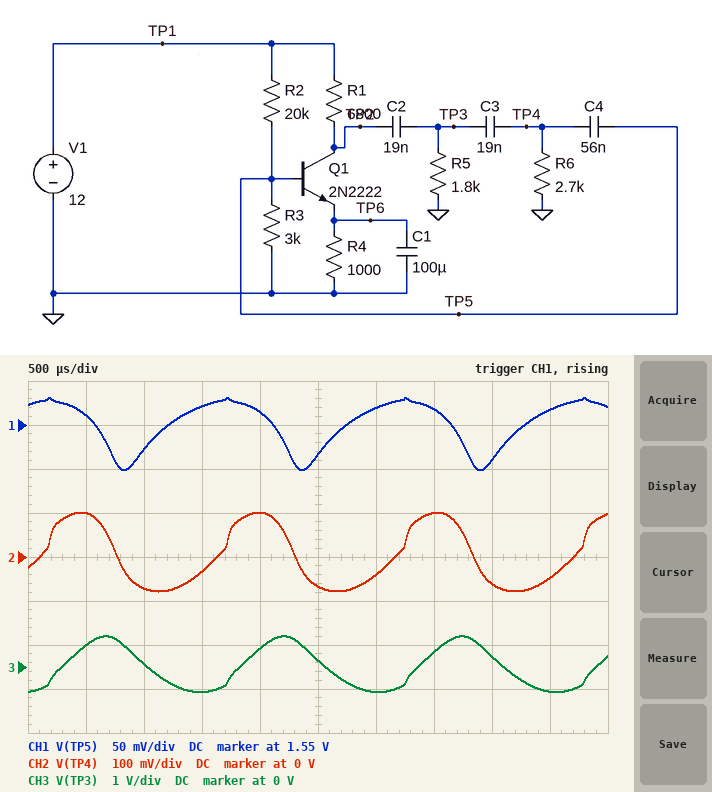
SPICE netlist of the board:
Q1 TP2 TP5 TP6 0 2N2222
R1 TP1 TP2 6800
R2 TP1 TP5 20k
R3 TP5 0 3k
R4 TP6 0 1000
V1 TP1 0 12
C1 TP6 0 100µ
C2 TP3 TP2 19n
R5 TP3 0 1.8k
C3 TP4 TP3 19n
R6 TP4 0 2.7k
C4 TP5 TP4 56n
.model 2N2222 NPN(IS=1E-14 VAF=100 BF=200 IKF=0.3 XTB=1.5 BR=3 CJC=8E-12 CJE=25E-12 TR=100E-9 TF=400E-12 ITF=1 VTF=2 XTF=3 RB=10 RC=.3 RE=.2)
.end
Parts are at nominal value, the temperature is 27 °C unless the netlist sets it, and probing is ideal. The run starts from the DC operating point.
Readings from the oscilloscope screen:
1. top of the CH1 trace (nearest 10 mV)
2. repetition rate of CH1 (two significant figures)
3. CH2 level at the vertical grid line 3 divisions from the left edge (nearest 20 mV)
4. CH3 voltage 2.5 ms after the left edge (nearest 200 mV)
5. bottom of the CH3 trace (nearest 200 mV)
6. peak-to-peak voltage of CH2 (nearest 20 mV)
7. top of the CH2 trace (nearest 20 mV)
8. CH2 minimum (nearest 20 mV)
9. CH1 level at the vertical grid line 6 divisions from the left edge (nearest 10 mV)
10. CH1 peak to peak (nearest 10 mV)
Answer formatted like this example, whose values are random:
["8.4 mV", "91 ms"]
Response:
["1.58 V", "650 Hz", "-40 mV", "200 mV", "-600 mV", "180 mV", "100 mV", "-80 mV", "1.57 V", "80 mV"]
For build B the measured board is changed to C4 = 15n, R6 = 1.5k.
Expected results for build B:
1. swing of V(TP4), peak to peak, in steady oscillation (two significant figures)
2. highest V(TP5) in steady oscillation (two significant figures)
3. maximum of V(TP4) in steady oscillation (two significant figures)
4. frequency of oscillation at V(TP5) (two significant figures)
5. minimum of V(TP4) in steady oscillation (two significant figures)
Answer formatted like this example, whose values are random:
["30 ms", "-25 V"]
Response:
["270 mV", "1.6 V", "140 mV", "1.1 kHz", "-130 mV"]
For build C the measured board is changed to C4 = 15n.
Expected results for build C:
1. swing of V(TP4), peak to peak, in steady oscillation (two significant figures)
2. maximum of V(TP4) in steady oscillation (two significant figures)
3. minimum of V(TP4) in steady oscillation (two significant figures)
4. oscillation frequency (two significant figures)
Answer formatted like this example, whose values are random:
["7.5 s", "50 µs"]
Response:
["390 mV", "210 mV", "-180 mV", "950 Hz"]
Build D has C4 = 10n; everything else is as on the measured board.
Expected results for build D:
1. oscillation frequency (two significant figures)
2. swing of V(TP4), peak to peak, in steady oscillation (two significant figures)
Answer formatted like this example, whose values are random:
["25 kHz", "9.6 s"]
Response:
["1.1 kHz", "410 mV"]
